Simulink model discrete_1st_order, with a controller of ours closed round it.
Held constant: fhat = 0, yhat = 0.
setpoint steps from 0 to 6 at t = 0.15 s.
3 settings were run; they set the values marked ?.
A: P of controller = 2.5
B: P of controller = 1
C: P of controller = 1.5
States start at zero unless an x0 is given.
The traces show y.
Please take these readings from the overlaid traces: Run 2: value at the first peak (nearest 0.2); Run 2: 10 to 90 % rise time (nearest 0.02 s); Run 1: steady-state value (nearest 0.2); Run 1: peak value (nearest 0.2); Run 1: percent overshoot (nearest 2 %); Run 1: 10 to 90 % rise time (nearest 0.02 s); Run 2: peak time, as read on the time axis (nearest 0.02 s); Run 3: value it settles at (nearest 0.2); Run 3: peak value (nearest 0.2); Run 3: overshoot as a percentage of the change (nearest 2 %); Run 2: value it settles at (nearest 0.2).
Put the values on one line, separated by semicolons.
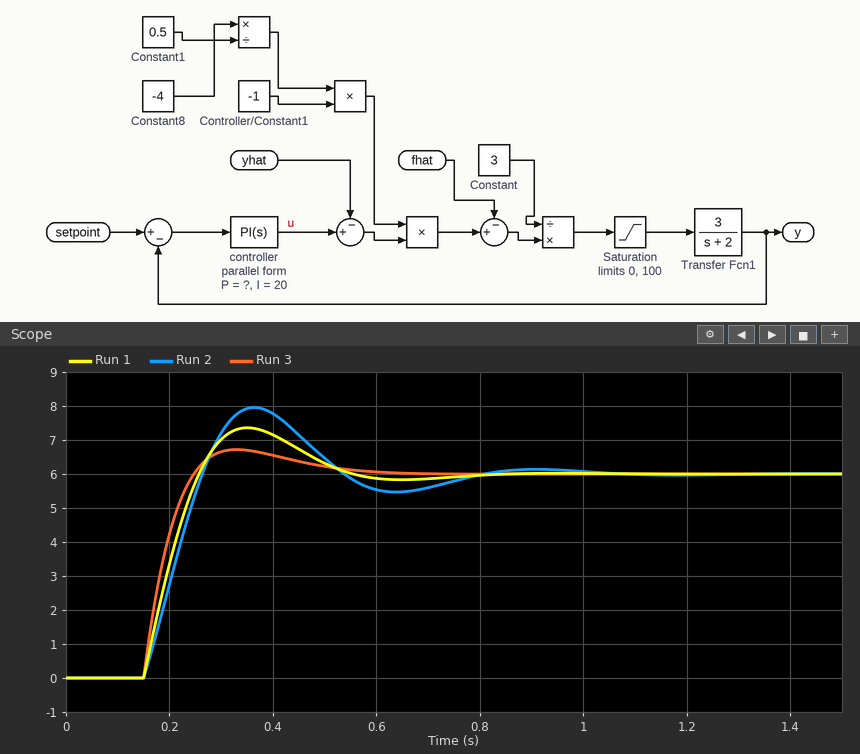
8.0; 0.08 s; 6.0; 7.4; 22 %; 0.08 s; 0.36 s; 6.0; 6.8; 12 %; 6.0
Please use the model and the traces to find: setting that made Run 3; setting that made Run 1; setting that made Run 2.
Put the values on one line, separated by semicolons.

A; C; B
